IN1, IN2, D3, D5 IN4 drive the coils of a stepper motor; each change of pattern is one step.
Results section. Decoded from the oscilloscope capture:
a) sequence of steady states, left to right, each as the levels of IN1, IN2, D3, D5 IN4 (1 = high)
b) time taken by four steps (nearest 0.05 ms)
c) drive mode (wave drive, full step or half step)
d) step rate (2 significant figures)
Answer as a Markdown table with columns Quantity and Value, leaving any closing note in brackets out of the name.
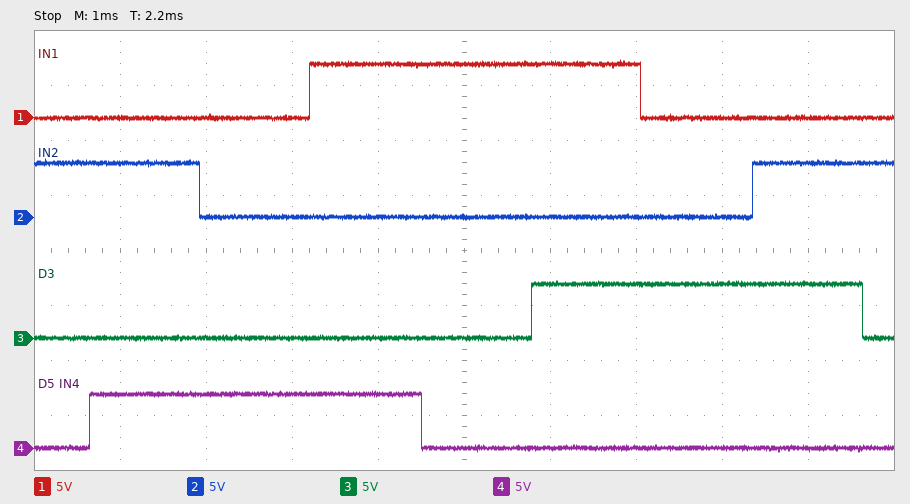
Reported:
| Quantity | Value |
|---|---|
| sequence of steady states, left to right, each as the levels of IN1, IN2, D3, D5 IN4 | 0100 0101 0001 1001 1000 1010 0010 0110 0100 |
| time taken by four steps | 5.15 ms |
| drive mode | half step |
| step rate | 780 steps/s |
